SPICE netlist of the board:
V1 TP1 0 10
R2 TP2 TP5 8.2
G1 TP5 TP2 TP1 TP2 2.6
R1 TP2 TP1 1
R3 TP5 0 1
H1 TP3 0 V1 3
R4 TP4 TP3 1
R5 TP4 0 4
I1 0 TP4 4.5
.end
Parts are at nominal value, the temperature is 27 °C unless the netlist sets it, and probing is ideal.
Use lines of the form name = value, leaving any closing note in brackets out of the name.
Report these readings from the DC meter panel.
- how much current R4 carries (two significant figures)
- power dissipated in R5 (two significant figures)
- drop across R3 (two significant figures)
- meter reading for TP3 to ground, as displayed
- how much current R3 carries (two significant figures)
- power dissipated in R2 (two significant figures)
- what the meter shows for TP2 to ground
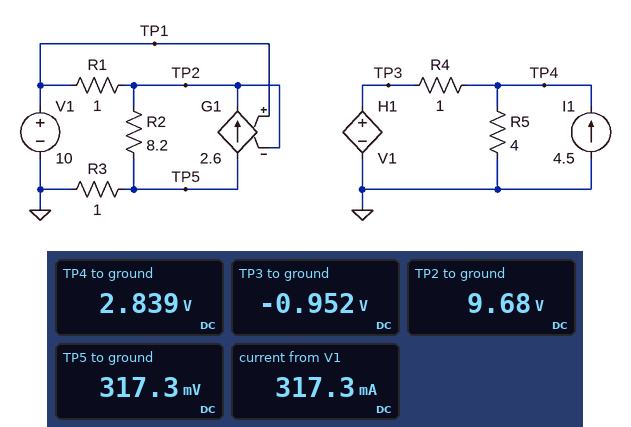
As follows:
how much current R4 carries = 3.8 A
power dissipated in R5 = 2.0 W
drop across R3 = 320 mV
meter reading for TP3 to ground, as displayed = -0.952 V
how much current R3 carries = 320 mA
power dissipated in R2 = 11 W
what the meter shows for TP2 to ground = 9.68 V
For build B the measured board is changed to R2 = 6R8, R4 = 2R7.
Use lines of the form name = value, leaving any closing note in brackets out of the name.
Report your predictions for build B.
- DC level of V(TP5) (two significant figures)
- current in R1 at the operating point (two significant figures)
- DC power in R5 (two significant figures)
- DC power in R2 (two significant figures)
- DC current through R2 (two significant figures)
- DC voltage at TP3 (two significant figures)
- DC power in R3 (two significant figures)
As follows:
DC level of V(TP5) = 380 mV
current in R1 at the operating point = 380 mA
DC power in R5 = 11 W
DC power in R2 = 13 W
DC current through R2 = 1.4 A
DC voltage at TP3 = -1.1 V
DC power in R3 = 140 mW
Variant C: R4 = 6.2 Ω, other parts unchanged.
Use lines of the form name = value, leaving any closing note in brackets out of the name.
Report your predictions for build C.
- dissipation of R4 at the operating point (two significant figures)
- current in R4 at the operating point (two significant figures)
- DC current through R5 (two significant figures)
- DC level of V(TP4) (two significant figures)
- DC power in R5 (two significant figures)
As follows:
dissipation of R4 at the operating point = 21 W
current in R4 at the operating point = 1.9 A
DC current through R5 = 2.6 A
DC level of V(TP4) = 11 V
DC power in R5 = 28 W
